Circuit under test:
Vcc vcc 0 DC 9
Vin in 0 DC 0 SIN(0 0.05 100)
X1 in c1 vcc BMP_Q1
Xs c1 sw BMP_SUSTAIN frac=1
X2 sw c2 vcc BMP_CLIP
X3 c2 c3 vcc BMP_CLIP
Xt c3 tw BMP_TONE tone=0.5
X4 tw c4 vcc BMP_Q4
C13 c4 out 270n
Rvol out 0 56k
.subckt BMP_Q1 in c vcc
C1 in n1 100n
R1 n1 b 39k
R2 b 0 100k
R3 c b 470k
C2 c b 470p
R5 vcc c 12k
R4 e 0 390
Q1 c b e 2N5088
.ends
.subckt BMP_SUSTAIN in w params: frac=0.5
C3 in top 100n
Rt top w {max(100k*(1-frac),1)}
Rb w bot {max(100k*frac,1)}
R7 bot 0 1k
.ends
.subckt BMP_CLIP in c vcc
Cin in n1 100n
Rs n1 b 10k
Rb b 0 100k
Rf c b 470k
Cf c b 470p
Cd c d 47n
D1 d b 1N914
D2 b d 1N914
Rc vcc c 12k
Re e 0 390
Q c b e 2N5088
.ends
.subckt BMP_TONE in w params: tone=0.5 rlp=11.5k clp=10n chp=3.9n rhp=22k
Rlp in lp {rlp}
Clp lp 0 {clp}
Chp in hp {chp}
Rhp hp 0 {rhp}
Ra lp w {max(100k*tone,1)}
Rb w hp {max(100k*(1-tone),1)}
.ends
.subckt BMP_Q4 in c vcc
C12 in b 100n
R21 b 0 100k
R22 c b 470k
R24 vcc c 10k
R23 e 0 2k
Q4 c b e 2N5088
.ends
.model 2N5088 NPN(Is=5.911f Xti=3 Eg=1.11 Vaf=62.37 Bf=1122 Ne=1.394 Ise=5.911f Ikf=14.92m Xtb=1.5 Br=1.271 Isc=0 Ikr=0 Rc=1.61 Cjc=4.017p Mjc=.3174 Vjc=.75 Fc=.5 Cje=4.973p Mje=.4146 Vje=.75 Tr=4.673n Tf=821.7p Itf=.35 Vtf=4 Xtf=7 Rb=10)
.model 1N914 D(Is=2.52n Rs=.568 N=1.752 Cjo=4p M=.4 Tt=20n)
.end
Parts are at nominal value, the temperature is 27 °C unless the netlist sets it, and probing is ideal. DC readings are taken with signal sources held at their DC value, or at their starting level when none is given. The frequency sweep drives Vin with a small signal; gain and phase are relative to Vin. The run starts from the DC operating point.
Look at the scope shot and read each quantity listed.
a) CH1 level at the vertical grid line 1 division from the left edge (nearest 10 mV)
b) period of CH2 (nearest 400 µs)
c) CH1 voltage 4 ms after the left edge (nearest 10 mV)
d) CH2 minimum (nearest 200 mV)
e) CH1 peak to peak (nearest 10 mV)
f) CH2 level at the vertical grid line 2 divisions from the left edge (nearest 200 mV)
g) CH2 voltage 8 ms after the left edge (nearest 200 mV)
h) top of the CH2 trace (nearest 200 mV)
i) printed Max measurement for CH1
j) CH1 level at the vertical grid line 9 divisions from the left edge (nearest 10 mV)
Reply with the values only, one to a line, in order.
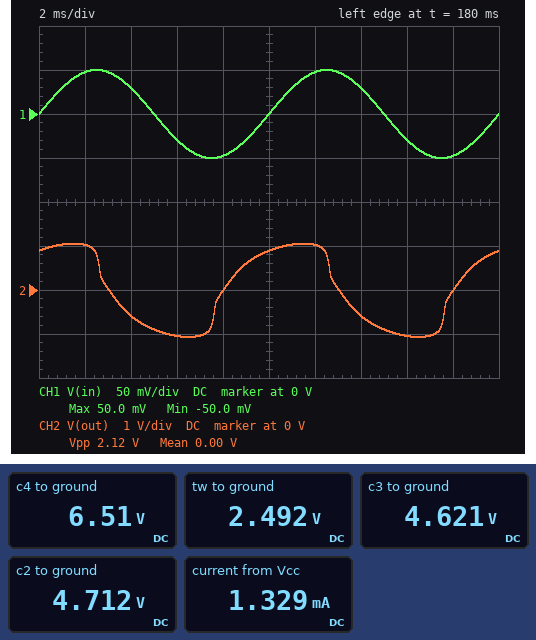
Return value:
50 mV
10.0 ms
30 mV
-1.0 V
100 mV
-600 mV
0 V
1.0 V
50.0 mV
-50 mV
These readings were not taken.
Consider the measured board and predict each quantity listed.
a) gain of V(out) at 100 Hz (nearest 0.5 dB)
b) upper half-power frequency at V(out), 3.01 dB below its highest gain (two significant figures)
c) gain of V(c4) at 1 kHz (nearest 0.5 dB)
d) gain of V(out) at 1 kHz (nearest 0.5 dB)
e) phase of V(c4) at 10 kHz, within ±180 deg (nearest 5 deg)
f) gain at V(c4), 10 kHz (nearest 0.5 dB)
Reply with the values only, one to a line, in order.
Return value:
55.0 dB
700 Hz
52.0 dB
52.0 dB
140 deg
16.0 dB
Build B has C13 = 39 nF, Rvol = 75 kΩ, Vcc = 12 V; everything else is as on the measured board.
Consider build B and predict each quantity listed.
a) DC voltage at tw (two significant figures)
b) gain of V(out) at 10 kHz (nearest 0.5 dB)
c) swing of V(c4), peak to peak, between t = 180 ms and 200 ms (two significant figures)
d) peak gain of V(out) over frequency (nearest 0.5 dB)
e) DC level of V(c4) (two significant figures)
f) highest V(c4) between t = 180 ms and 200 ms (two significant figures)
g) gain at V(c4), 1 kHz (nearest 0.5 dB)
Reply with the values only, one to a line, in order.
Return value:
2.8 V
17.0 dB
2.5 V
59.0 dB
8.2 V
9.4 V
53.0 dB
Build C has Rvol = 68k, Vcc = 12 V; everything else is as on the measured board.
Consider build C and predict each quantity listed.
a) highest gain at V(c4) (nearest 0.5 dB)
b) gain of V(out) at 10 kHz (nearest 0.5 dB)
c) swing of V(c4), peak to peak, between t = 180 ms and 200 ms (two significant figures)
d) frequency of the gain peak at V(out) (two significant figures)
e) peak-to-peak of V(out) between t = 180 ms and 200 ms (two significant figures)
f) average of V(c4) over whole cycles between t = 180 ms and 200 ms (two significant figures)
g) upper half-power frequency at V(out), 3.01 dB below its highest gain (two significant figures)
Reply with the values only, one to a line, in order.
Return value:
59.0 dB
17.0 dB
2.4 V
260 Hz
2.3 V
8.2 V
690 Hz
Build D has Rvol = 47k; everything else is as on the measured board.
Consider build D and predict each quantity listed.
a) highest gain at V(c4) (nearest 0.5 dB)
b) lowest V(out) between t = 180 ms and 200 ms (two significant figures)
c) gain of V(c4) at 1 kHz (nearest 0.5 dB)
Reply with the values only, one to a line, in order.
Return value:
57.5 dB
-1.0 V
51.5 dB
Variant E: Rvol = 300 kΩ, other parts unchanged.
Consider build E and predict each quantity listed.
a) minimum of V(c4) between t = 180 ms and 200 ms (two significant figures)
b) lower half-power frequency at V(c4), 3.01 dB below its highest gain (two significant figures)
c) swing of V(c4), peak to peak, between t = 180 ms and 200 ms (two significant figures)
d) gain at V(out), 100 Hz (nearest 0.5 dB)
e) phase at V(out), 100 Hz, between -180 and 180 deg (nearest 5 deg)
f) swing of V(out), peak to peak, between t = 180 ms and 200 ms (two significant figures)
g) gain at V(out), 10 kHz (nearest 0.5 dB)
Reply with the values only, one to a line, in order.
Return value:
5.3 V
95 Hz
2.5 V
56.0 dB
90 deg
2.4 V
17.0 dB
